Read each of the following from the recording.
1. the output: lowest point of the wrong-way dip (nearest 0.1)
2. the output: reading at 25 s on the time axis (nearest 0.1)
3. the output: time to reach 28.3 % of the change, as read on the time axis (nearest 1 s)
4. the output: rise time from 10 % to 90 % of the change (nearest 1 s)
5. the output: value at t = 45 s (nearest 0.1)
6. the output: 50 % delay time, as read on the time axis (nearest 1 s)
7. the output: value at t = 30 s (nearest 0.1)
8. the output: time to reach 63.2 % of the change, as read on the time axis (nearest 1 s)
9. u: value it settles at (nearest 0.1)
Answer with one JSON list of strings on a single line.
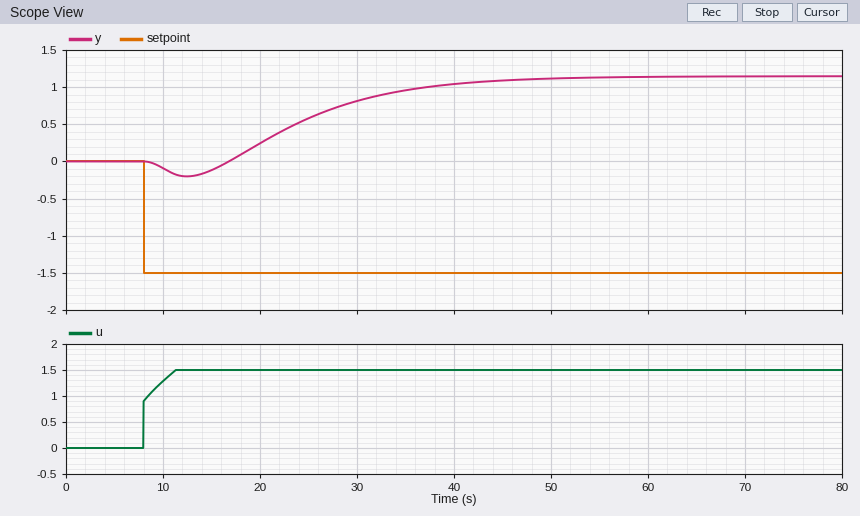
["-0.2", "0.6", "21 s", "21 s", "1.1", "25 s", "0.8", "28 s", "1.5"]
